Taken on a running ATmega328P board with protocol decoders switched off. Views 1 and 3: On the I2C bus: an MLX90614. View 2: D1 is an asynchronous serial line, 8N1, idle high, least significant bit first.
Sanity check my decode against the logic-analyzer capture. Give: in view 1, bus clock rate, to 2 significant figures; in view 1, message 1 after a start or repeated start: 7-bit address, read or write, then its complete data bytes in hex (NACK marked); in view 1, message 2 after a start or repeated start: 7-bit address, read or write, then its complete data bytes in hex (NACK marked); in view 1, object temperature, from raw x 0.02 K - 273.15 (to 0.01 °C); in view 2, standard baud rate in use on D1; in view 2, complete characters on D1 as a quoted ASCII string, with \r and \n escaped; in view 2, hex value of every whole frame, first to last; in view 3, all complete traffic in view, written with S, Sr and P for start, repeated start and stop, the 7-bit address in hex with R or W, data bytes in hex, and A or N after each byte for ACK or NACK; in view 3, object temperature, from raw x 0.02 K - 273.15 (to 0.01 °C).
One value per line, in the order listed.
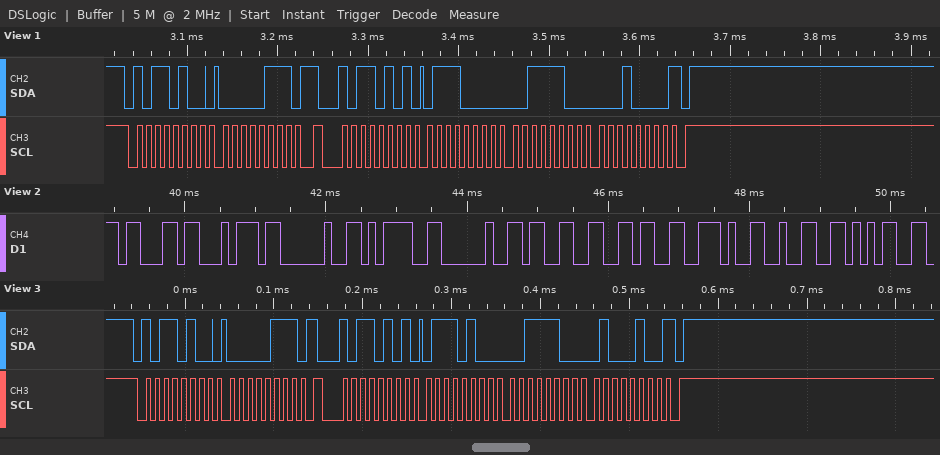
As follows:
100 kHz
0x5A write: 07
0x5A read: 70 3C 10 NACK
36.29 °C
9600 baud
"ct = 36.25"
63 74 20 3D 20 33 36 2E 32 35
S 5AW A 07 A Sr 5AR A 74 A 3C A 44 N P
36.37 °C
